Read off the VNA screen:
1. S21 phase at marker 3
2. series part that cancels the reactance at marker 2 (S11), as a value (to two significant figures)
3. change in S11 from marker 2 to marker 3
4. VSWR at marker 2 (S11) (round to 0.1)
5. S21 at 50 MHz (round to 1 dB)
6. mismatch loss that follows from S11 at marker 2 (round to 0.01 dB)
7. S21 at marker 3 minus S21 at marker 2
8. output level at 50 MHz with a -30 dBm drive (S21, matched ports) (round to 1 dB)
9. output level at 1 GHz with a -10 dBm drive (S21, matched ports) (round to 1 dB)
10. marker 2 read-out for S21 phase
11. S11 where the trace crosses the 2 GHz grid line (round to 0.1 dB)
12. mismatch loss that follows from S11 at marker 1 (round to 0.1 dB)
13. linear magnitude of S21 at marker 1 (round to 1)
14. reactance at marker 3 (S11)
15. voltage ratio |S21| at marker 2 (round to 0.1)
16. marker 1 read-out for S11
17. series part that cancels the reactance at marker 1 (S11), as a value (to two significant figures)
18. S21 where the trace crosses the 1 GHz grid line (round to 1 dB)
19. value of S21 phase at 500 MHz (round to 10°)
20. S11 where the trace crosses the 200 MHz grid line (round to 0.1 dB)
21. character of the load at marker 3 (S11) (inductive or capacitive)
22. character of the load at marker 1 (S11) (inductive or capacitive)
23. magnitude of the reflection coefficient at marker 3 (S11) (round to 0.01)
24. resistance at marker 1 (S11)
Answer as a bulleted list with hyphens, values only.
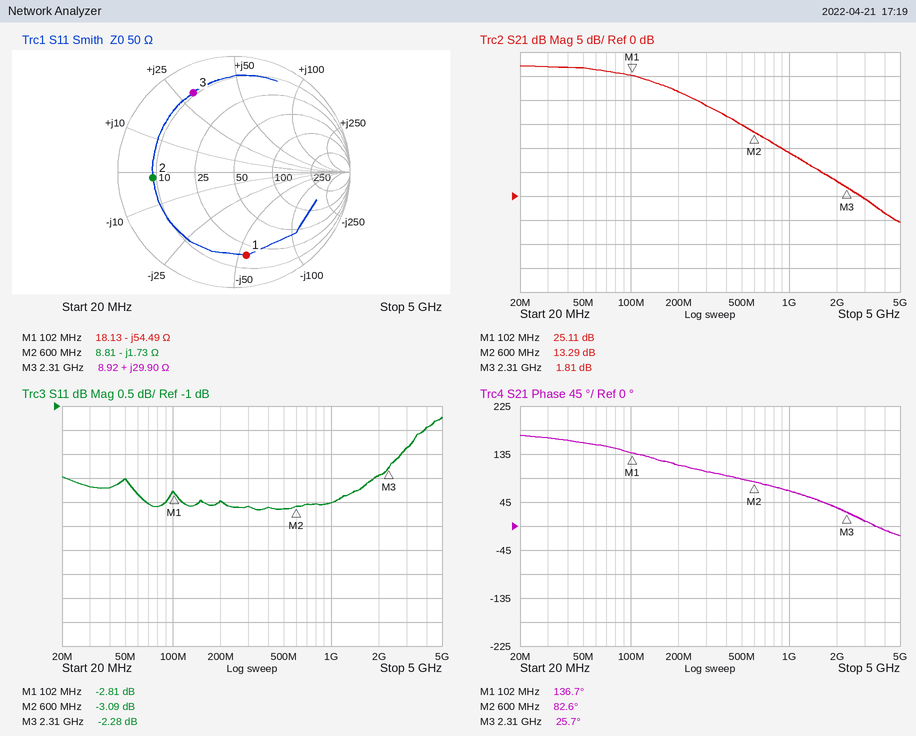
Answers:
- 25.7°
- 460 pH
- 0.81 dB
- 5.7
- 27 dB
- 2.93 dB
- -11.48 dB
- -3 dBm
- -1 dBm
- 82.6°
- -2.4 dB
- 3.2 dB
- 18
- +29.90 Ω
- 4.6
- -2.81 dB
- 85 nH
- 9 dB
- 90°
- -3.0 dB
- inductive
- capacitive
- 0.77
- 18.13 Ω
